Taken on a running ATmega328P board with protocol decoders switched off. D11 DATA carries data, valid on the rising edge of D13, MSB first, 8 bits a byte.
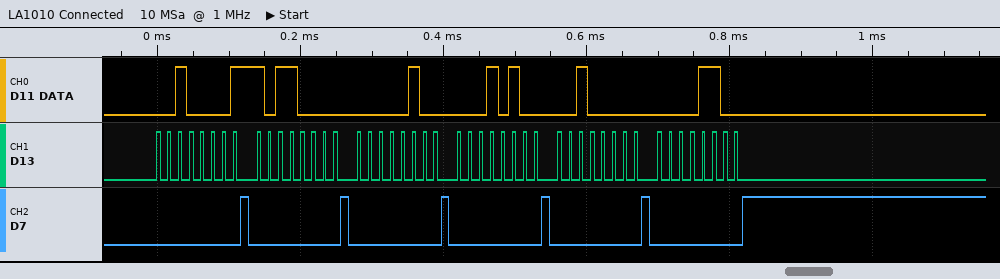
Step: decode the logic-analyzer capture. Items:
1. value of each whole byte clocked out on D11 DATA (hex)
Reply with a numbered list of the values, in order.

1. 0x21 0xB0 0x04 0x14 0x20 0x0C
